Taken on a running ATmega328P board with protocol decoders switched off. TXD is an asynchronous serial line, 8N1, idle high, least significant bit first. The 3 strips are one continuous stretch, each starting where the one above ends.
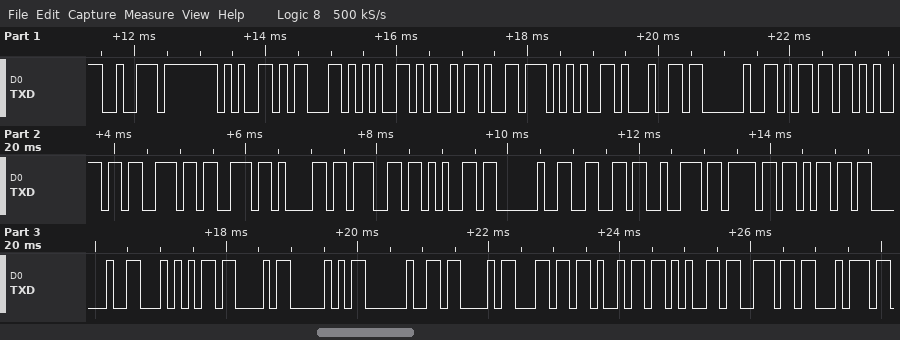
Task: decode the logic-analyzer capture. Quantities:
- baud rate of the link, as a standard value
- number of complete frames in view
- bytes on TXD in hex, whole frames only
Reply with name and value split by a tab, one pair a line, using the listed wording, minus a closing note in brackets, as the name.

baud rate of the link, as a standard value	9600 baud
number of complete frames in view	32
bytes on TXD in hex, whole frames only	0x72 0x65 0x63 0x65 0x69 0x76 0x65 0x64 0x20 0x6D 0x65 0x73 0x73 0x61 0x67 0x65 0x20 0x66 0x72 0x6F 0x6D 0x20 0x54 0x43 0x50 0x20 0x43 0x6C 0x69 0x65 0x6E 0x74
